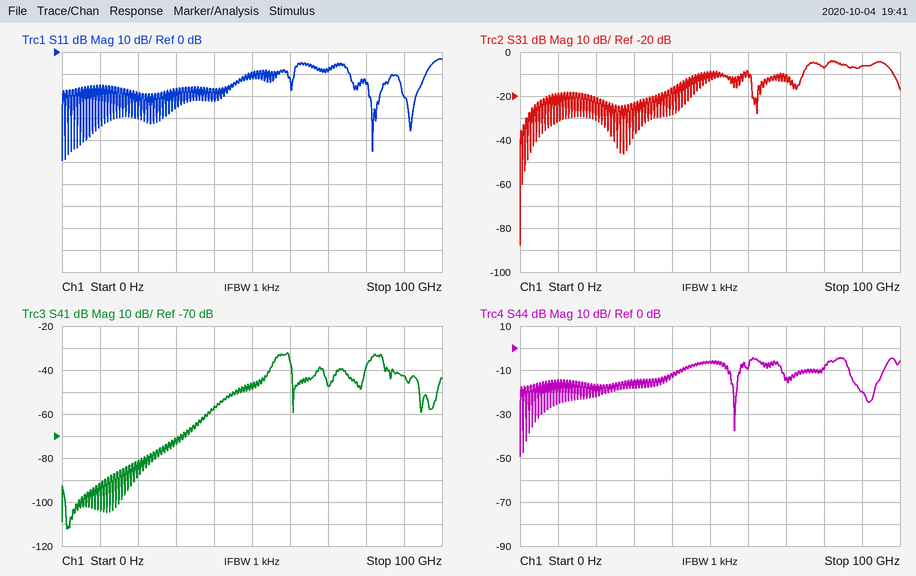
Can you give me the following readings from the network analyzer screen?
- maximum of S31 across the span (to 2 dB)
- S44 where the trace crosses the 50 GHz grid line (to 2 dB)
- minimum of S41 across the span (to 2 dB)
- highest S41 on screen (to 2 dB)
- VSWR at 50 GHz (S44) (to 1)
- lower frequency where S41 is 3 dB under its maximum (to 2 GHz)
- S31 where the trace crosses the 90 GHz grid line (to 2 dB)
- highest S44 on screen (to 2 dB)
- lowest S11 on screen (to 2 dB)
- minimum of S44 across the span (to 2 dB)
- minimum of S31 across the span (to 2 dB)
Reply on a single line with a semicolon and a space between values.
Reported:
-4 dB; -6 dB; -112 dB; -32 dB; 3; 56 GHz; -6 dB; -4 dB; -50 dB; -50 dB; -88 dB
